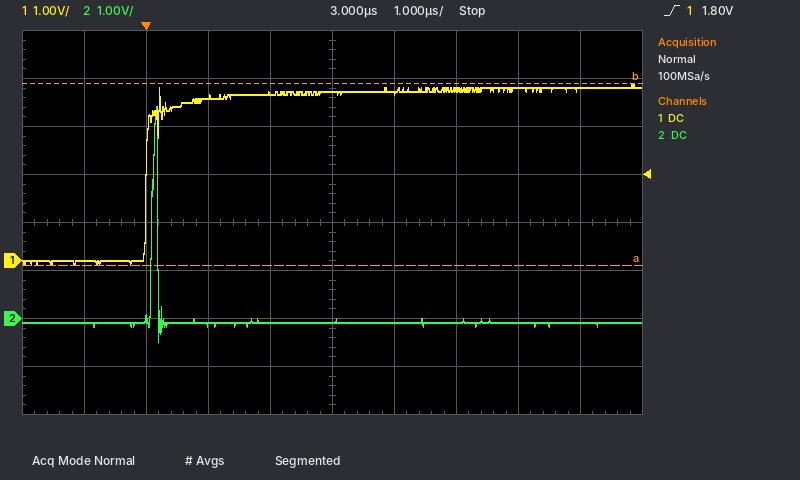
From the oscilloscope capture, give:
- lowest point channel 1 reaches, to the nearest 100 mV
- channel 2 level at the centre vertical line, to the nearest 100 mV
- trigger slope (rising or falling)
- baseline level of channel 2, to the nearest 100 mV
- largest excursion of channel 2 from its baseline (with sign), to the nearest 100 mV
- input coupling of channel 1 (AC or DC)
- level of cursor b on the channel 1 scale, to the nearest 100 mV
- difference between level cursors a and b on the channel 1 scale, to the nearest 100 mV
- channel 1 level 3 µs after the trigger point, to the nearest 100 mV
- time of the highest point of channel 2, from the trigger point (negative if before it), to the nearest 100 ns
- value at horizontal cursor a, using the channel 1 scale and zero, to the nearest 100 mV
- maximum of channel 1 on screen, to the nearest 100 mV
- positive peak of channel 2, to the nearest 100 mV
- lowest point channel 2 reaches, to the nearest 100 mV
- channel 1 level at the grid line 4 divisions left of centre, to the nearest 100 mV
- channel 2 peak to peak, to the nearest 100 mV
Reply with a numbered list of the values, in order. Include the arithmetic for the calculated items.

1. -100 mV
2. -100 mV
3. rising
4. -100 mV
5. 4.4 V − (-100 mV) = +4.5 V
6. DC
7. 3.7 V
8. 3.8 V
9. 3.5 V
10. +200 ns
11. -100 mV
12. 3.7 V
13. 4.4 V
14. -500 mV
15. 0.0 V
16. 4.4 V − (-500 mV) = 4.9 V
